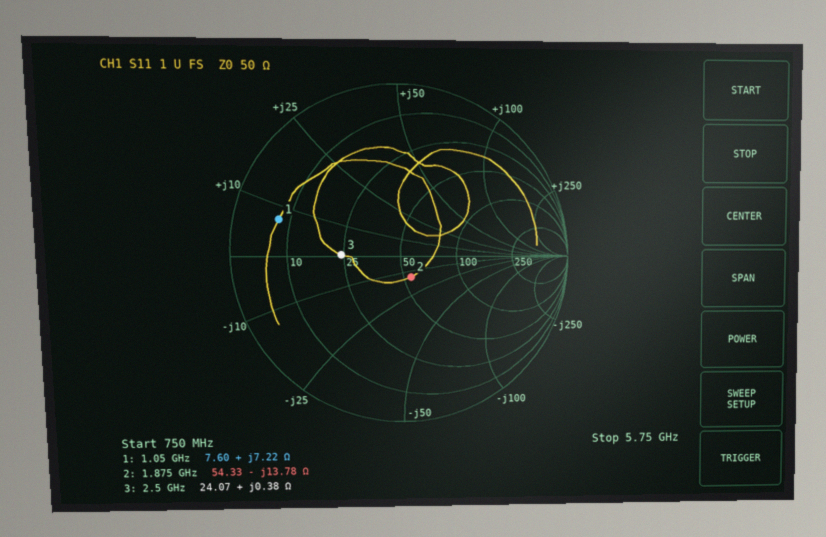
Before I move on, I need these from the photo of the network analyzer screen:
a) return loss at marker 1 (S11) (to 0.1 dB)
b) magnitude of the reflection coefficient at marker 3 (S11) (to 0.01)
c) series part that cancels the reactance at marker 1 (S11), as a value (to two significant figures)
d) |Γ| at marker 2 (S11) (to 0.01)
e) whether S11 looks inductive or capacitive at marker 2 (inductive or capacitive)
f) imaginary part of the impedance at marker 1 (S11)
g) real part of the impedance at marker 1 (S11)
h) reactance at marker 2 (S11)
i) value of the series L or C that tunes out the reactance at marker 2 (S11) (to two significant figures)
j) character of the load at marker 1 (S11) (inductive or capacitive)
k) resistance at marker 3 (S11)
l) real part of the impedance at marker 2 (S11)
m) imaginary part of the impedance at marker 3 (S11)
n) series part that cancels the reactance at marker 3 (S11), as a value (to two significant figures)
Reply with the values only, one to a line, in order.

2.6 dB
0.35
21 pF
0.14
capacitive
+7.22 Ω
7.60 Ω
-13.78 Ω
1.2 nH
inductive
24.07 Ω
54.33 Ω
+0.38 Ω
170 pF
